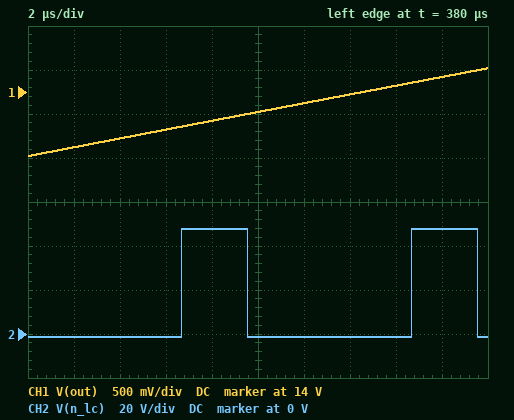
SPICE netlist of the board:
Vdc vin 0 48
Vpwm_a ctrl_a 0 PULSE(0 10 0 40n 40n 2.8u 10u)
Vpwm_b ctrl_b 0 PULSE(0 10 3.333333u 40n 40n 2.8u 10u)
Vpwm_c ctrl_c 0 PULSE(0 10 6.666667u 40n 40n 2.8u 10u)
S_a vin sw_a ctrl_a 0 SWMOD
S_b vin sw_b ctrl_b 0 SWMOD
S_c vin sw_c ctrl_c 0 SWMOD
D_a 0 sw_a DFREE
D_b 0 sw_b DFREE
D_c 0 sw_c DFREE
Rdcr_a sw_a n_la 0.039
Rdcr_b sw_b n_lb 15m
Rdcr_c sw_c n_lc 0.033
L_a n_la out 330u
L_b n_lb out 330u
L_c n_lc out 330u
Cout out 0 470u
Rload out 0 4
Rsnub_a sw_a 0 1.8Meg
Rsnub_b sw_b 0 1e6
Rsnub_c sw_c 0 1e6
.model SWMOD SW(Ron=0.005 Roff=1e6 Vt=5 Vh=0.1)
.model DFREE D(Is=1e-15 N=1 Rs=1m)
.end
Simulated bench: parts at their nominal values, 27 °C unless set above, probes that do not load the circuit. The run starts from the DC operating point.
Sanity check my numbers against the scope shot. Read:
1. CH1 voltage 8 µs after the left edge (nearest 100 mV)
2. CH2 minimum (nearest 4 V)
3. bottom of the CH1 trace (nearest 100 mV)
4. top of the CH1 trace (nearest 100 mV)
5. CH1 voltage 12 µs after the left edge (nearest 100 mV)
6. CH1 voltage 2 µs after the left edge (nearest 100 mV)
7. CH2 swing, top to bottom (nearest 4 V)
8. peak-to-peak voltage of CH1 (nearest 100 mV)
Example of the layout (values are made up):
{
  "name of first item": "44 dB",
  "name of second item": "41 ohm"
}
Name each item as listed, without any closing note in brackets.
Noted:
{
  "CH1 voltage 8 µs after the left edge": "13.7 V",
  "CH2 minimum": "0 V",
  "bottom of the CH1 trace": "13.3 V",
  "top of the CH1 trace": "14.3 V",
  "CH1 voltage 12 µs after the left edge": "13.9 V",
  "CH1 voltage 2 µs after the left edge": "13.4 V",
  "CH2 swing, top to bottom": "48 V",
  "peak-to-peak voltage of CH1": "1.0 V"
}
